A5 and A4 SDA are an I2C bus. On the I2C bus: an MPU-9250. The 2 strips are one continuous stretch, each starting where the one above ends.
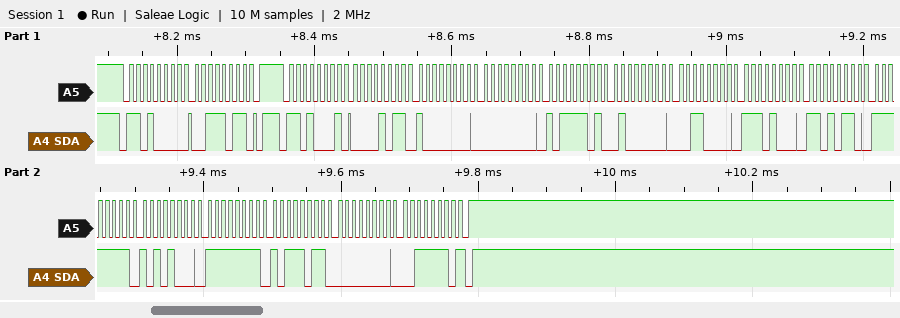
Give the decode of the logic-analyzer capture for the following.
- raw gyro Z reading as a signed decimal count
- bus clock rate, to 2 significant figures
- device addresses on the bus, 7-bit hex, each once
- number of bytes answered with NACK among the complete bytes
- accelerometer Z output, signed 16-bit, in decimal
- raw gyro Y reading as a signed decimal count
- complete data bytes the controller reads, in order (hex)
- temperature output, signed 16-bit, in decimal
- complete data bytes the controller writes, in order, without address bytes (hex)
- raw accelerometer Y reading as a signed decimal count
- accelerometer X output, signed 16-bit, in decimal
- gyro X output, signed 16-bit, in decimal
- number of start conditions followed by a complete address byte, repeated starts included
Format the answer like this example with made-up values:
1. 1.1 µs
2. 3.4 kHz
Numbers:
1. 62
2. 100 kHz
3. 0x68
4. 1
5. 16432
6. -69
7. 0B 80 00 BD 40 30 E8 D6 FF A8 FF BB 00 3E
8. -5930
9. 3B
10. 189
11. 2944
12. -88
13. 2
